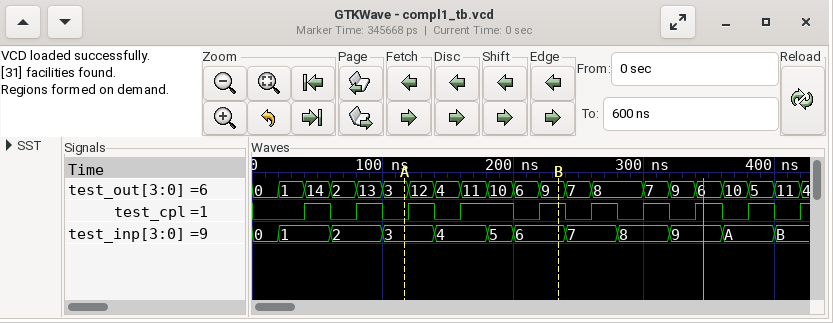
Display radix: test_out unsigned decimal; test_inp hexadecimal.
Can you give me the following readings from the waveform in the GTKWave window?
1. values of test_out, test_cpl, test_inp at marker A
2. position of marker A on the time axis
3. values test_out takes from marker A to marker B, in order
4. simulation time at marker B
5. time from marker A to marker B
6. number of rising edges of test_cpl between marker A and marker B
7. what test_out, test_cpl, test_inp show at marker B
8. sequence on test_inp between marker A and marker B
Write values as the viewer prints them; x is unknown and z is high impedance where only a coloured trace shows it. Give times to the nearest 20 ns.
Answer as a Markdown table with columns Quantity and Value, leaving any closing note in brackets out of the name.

| Quantity | Value |
|---|---|
| values of test_out, test_cpl, test_inp at marker A | test_out=3, test_cpl=0, test_inp=3 |
| position of marker A on the time axis | 120 ns |
| values test_out takes from marker A to marker B, in order | 3, 12, 4, 11, 10, 6, 9 |
| simulation time at marker B | 240 ns |
| time from marker A to marker B | 120 ns |
| number of rising edges of test_cpl between marker A and marker B | 3 |
| what test_out, test_cpl, test_inp show at marker B | test_out=9, test_cpl=1, test_inp=6 |
| sequence on test_inp between marker A and marker B | 3, 4, 5, 6 |
